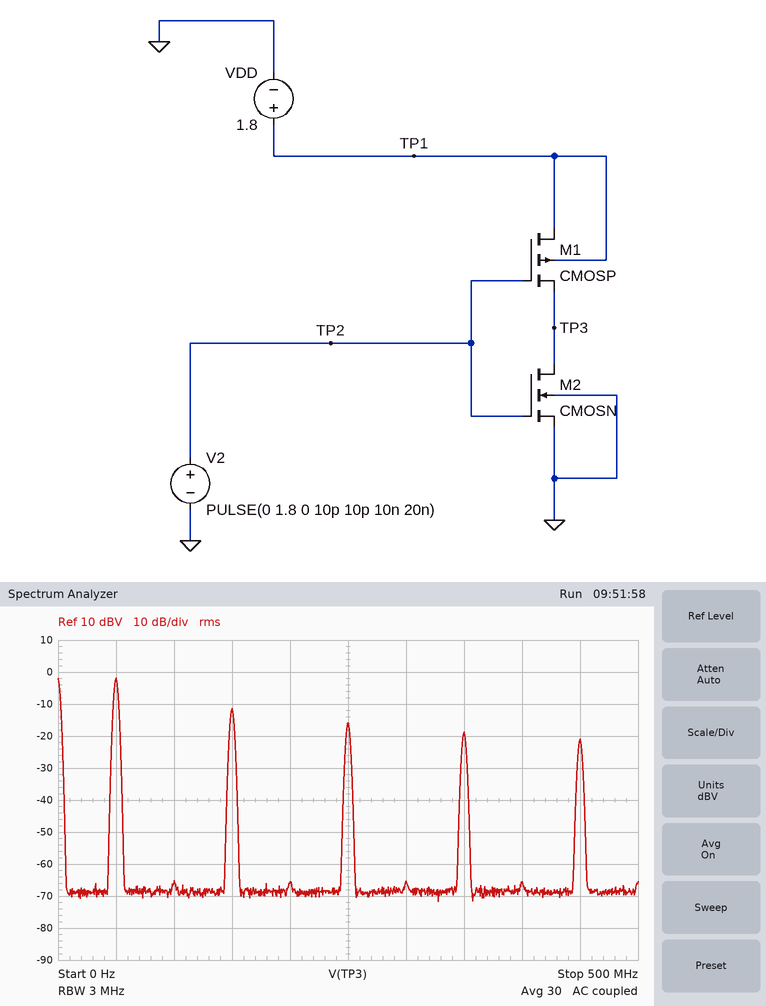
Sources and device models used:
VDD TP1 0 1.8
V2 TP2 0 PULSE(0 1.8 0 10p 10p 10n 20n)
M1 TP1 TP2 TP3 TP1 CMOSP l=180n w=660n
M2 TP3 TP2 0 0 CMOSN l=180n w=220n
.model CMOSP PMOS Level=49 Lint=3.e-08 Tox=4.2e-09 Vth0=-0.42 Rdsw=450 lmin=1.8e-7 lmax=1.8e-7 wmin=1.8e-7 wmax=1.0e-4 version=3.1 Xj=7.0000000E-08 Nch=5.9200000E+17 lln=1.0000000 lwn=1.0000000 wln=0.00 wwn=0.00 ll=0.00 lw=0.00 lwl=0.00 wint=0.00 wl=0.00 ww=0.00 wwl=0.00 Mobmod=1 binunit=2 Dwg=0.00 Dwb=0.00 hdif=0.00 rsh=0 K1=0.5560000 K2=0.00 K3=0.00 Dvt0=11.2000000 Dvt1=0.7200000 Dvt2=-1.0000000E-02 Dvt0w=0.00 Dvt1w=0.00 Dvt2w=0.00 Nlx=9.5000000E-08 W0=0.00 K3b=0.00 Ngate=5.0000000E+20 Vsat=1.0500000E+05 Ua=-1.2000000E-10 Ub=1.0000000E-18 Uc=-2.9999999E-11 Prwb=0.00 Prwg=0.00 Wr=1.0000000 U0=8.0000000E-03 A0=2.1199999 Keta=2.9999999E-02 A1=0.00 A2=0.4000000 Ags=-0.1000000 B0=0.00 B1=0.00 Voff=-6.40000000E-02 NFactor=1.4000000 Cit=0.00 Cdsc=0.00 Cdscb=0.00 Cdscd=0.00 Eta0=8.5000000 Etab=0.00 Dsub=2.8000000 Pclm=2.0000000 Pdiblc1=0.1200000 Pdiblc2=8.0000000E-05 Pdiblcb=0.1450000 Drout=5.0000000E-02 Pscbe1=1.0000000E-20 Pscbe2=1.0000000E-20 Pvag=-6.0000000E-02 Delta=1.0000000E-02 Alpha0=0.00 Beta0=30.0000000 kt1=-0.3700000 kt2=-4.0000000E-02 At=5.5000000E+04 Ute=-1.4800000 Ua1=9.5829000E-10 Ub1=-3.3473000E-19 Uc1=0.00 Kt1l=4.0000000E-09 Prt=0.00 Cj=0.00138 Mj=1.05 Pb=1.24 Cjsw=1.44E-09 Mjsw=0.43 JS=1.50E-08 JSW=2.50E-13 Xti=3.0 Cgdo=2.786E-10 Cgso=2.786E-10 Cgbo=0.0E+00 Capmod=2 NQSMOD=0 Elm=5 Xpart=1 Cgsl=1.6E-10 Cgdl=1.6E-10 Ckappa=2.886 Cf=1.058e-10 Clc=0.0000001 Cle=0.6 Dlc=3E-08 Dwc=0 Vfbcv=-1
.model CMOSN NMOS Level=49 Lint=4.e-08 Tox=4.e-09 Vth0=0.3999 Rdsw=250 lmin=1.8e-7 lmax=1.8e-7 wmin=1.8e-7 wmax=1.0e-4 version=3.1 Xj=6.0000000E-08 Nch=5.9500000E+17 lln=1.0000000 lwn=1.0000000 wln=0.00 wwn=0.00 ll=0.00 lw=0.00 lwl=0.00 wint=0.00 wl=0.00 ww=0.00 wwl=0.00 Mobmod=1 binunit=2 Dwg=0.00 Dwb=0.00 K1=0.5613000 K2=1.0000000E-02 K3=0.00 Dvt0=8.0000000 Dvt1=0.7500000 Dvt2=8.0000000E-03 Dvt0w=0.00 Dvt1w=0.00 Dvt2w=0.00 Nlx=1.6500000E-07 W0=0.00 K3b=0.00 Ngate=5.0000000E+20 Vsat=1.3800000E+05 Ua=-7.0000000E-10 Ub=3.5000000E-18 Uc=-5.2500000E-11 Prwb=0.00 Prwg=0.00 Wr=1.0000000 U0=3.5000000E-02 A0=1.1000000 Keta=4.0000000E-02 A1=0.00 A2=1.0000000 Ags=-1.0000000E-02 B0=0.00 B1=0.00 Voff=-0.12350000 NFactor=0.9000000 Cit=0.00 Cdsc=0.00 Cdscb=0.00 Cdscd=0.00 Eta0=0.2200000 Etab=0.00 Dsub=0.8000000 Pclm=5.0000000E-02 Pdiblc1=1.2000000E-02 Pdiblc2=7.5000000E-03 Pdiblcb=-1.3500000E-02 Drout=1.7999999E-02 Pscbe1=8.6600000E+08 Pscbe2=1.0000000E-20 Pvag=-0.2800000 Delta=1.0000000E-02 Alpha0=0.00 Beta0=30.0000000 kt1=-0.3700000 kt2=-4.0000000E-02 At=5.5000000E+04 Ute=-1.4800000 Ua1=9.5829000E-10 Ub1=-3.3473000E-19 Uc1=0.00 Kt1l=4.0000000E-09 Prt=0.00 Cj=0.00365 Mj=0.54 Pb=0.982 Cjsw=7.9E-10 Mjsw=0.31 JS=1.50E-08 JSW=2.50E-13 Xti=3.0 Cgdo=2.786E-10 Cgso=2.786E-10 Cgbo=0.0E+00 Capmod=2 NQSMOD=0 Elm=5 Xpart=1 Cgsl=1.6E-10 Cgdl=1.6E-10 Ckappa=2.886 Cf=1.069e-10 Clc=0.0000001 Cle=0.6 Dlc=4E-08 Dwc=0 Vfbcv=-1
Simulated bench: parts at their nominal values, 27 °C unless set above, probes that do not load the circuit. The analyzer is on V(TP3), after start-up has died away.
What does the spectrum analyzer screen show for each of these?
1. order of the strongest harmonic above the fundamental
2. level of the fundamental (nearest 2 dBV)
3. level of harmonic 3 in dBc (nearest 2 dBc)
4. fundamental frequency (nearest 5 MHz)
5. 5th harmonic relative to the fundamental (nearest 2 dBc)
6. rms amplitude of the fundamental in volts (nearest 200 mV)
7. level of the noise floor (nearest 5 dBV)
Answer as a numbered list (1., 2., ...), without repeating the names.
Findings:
1. 3
2. -2 dBV
3. -10 dBc
4. 50 MHz
5. -14 dBc
6. 800 mV
7. -70 dBV
